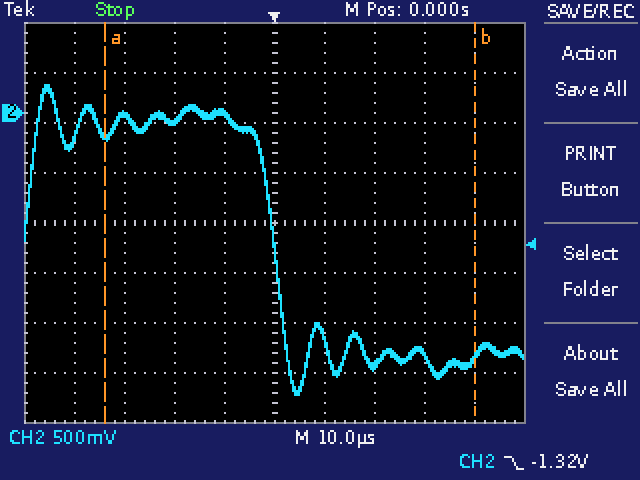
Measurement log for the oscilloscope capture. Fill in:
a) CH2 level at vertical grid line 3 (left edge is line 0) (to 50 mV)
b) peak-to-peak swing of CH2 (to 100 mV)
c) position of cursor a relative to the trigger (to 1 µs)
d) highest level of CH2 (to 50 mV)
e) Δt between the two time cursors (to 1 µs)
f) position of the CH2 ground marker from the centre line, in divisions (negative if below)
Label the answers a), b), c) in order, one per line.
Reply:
a) -100 mV
b) 3.10 V
c) -34 µs
d) 300 mV
e) 74 µs
f) +2.2 div
